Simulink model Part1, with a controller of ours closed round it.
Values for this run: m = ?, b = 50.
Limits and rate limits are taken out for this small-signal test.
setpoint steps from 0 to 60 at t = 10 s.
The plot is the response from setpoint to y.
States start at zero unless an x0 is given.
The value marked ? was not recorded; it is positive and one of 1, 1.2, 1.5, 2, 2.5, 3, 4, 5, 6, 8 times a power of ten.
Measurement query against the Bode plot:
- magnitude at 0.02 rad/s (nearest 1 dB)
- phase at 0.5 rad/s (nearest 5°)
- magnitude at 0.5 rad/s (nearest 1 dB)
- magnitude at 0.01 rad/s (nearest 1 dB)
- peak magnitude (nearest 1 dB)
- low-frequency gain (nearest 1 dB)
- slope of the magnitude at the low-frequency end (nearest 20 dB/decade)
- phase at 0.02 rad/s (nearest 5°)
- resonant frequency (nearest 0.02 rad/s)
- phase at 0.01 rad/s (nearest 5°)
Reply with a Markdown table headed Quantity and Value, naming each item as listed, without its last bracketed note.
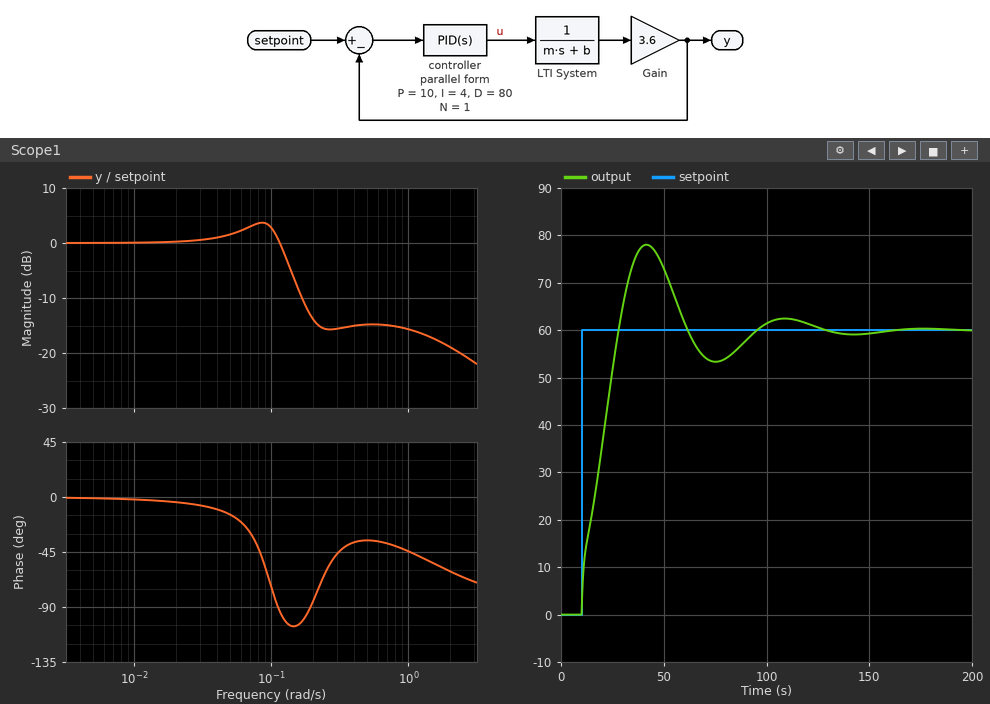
| Quantity | Value |
|---|---|
| magnitude at 0.02 rad/s | 0 dB |
| phase at 0.5 rad/s | -35° |
| magnitude at 0.5 rad/s | -15 dB |
| magnitude at 0.01 rad/s | 0 dB |
| peak magnitude | 4 dB |
| low-frequency gain | 0 dB |
| slope of the magnitude at the low-frequency end | 0 dB/decade |
| phase at 0.02 rad/s | -5° |
| resonant frequency | 0.08 rad/s |
| phase at 0.01 rad/s | 0° |
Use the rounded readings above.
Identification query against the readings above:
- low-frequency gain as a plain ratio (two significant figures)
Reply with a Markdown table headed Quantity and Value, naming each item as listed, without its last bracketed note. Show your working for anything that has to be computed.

| Quantity | Value |
|---|---|
| low-frequency gain as a plain ratio | 10^(0 / 20) = 1.0 |
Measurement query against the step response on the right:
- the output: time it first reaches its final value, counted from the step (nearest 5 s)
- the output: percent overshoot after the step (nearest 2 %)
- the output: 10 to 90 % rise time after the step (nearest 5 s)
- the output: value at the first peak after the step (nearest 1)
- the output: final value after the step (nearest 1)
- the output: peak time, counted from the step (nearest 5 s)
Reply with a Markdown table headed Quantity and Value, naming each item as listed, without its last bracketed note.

| Quantity | Value |
|---|---|
| the output: time it first reaches its final value, counted from the step | 20 s |
| the output: percent overshoot after the step | 30 % |
| the output: 10 to 90 % rise time after the step | 15 s |
| the output: value at the first peak after the step | 78 |
| the output: final value after the step | 60 |
| the output: peak time, counted from the step | 30 s |
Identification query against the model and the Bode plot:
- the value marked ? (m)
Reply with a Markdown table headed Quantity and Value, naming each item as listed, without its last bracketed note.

| Quantity | Value |
|---|---|
| the value marked ? | 1200 |
